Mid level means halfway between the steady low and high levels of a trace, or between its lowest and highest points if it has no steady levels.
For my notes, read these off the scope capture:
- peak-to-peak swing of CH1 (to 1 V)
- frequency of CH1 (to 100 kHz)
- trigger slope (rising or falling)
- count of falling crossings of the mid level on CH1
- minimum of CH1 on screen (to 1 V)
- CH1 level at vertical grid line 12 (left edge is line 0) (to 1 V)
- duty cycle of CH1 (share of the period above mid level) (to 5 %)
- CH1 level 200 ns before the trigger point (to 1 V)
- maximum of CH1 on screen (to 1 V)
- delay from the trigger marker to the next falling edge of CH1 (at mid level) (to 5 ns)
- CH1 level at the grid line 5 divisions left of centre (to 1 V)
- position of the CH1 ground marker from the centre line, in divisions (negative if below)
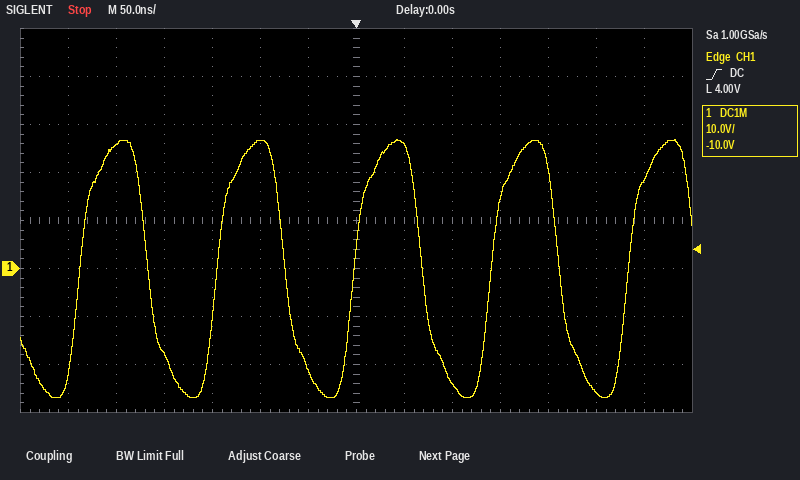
54 V
7.0 MHz
rising
4
-27 V
-26 V
50 %
-18 V
27 V
70 ns
26 V
-1.0 div
